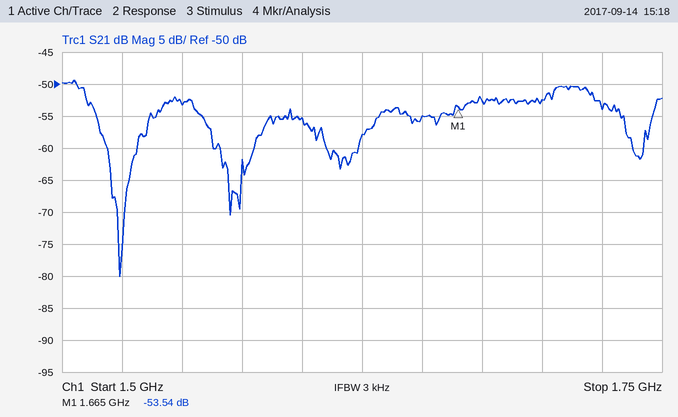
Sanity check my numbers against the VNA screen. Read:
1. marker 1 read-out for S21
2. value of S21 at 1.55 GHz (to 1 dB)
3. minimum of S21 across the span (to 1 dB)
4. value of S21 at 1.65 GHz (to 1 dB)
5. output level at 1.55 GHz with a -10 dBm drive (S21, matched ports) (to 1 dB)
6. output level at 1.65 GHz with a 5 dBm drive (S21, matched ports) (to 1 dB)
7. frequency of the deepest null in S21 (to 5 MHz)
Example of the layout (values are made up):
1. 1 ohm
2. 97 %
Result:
1. -53.54 dB
2. -53 dB
3. -80 dB
4. -55 dB
5. -63 dBm
6. -50 dBm
7. 1.525 GHz
